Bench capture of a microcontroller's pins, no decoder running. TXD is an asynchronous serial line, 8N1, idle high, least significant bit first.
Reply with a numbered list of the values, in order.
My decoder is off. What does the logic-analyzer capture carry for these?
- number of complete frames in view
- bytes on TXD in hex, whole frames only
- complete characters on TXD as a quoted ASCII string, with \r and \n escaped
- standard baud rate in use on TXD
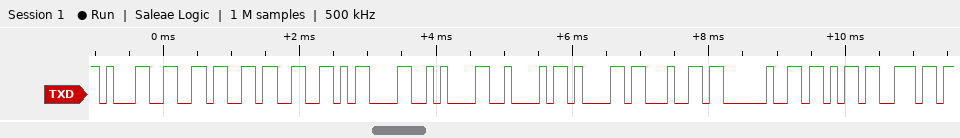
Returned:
1. 11
2. 31 36 33 0D 0A 42 61 64 20 6B 6E
3. "163\r\nBad kn"
4. 9600 baud
